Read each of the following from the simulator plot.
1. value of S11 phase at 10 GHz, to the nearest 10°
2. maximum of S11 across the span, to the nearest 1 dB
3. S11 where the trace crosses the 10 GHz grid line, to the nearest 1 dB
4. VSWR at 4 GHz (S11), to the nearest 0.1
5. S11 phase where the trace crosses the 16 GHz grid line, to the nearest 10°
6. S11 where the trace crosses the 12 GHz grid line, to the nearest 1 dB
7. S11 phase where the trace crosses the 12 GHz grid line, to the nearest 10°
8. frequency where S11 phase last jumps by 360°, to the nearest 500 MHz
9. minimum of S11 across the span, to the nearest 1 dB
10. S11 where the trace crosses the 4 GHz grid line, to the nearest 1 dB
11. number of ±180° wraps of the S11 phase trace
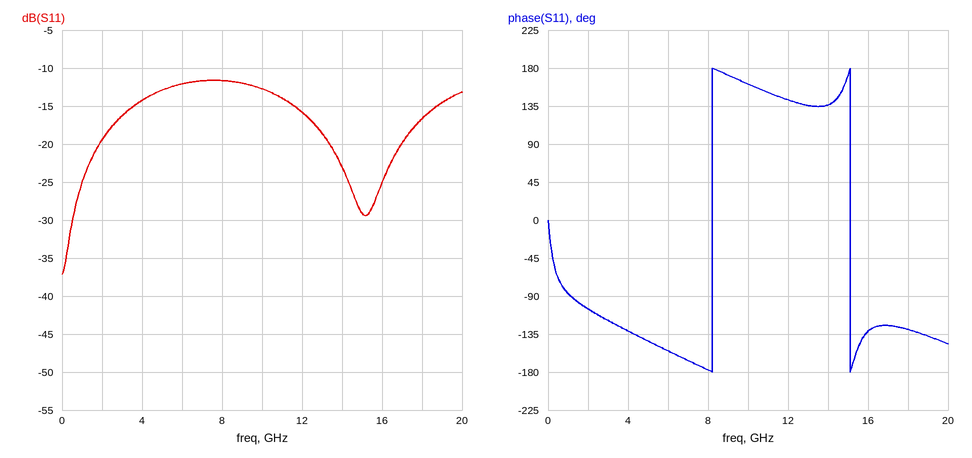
160°
-12 dB
-13 dB
1.5
-130°
-16 dB
140°
15.0 GHz
-37 dB
-14 dB
2
